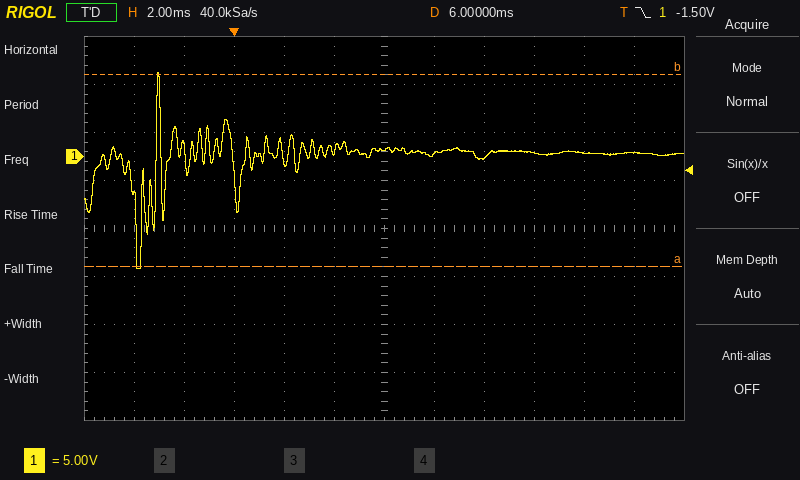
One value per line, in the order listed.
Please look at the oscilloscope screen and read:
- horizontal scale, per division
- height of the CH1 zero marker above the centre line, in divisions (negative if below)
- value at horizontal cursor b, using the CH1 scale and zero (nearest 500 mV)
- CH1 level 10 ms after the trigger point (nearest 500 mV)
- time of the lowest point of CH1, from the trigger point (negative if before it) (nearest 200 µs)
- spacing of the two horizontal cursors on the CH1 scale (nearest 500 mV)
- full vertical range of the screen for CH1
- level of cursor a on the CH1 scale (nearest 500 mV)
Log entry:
2 ms
+1.5 div
8.5 V
0.0 V
-3.8 ms
20.0 V
40 V
-11.5 V
